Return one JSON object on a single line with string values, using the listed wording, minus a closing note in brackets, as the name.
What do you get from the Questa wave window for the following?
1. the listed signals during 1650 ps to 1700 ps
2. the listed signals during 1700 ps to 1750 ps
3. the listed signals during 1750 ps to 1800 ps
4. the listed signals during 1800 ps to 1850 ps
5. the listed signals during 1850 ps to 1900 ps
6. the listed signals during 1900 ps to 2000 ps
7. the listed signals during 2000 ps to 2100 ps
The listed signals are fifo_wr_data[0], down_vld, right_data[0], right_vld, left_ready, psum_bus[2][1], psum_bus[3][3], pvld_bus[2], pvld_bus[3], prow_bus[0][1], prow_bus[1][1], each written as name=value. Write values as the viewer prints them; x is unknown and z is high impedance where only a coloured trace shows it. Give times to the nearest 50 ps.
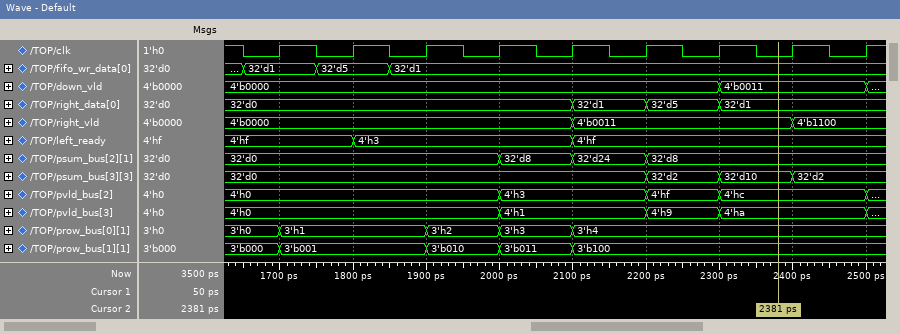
{"the listed signals during 1650 ps to 1700 ps": "fifo_wr_data[0]=32'd1, down_vld=4'b0000, right_data[0]=32'd0, right_vld=4'b0000, left_ready=4'hf, psum_bus[2][1]=32'd0, psum_bus[3][3]=32'd0, pvld_bus[2]=4'h0, pvld_bus[3]=4'h0, prow_bus[0][1]=3'h0, prow_bus[1][1]=3'b000", "the listed signals during 1700 ps to 1750 ps": "fifo_wr_data[0]=32'd1, down_vld=4'b0000, right_data[0]=32'd0, right_vld=4'b0000, left_ready=4'hf, psum_bus[2][1]=32'd0, psum_bus[3][3]=32'd0, pvld_bus[2]=4'h0, pvld_bus[3]=4'h0, prow_bus[0][1]=3'h1, prow_bus[1][1]=3'b001", "the listed signals during 1750 ps to 1800 ps": "fifo_wr_data[0]=32'd5, down_vld=4'b0000, right_data[0]=32'd0, right_vld=4'b0000, left_ready=4'hf, psum_bus[2][1]=32'd0, psum_bus[3][3]=32'd0, pvld_bus[2]=4'h0, pvld_bus[3]=4'h0, prow_bus[0][1]=3'h1, prow_bus[1][1]=3'b001", "the listed signals during 1800 ps to 1850 ps": "fifo_wr_data[0]=32'd5, down_vld=4'b0000, right_data[0]=32'd0, right_vld=4'b0000, left_ready=4'h3, psum_bus[2][1]=32'd0, psum_bus[3][3]=32'd0, pvld_bus[2]=4'h0, pvld_bus[3]=4'h0, prow_bus[0][1]=3'h1, prow_bus[1][1]=3'b001", "the listed signals during 1850 ps to 1900 ps": "fifo_wr_data[0]=32'd1, down_vld=4'b0000, right_data[0]=32'd0, right_vld=4'b0000, left_ready=4'h3, psum_bus[2][1]=32'd0, psum_bus[3][3]=32'd0, pvld_bus[2]=4'h0, pvld_bus[3]=4'h0, prow_bus[0][1]=3'h1, prow_bus[1][1]=3'b001", "the listed signals during 1900 ps to 2000 ps": "fifo_wr_data[0]=32'd1, down_vld=4'b0000, right_data[0]=32'd0, right_vld=4'b0000, left_ready=4'h3, psum_bus[2][1]=32'd0, psum_bus[3][3]=32'd0, pvld_bus[2]=4'h0, pvld_bus[3]=4'h0, prow_bus[0][1]=3'h2, prow_bus[1][1]=3'b010", "the listed signals during 2000 ps to 2100 ps": "fifo_wr_data[0]=32'd1, down_vld=4'b0000, right_data[0]=32'd0, right_vld=4'b0000, left_ready=4'h3, psum_bus[2][1]=32'd8, psum_bus[3][3]=32'd0, pvld_bus[2]=4'h3, pvld_bus[3]=4'h1, prow_bus[0][1]=3'h3, prow_bus[1][1]=3'b011"}
